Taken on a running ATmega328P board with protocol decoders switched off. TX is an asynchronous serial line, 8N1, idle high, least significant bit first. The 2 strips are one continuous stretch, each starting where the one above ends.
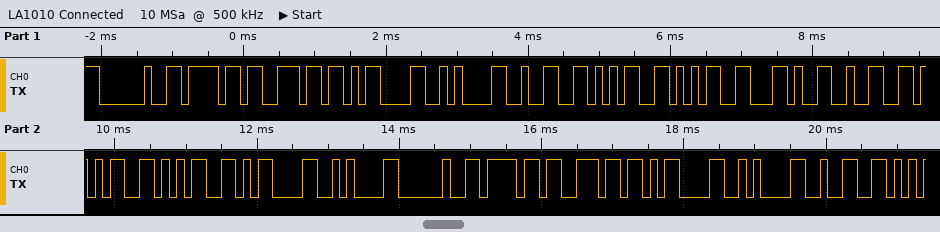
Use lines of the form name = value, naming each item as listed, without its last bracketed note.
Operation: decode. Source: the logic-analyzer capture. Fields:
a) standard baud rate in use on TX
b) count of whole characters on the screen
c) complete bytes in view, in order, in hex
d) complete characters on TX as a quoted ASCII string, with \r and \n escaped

standard baud rate in use on TX = 9600 baud
count of whole characters on the screen = 20
complete bytes in view, in order, in hex = 20 6F 6E 0D 0A 32 35 35 2C 32 35 35 0D 0A 20 6F 6E 0D 0A 32
complete characters on TX as a quoted ASCII string, with \r and \n escaped = " on\r\n255,255\r\n on\r\n2"
